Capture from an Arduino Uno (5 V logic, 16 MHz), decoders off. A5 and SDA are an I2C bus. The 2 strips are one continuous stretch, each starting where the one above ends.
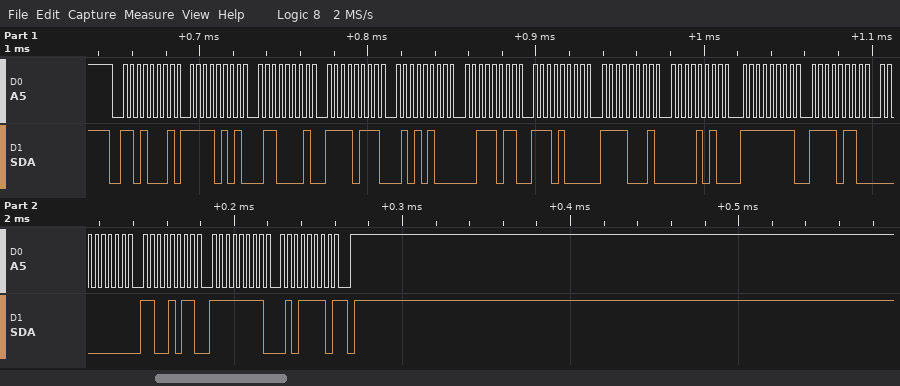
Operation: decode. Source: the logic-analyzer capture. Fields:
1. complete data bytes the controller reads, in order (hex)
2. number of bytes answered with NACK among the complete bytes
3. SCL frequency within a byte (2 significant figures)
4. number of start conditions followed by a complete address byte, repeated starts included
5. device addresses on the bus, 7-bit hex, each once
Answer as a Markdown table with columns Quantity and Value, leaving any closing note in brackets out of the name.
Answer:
| Quantity | Value |
|---|---|
| complete data bytes the controller reads, in order | F5 61 F7 54 3B E8 F1 0A FF F6 00 CB FF 5E |
| number of bytes answered with NACK among the complete bytes | 1 |
| SCL frequency within a byte | 250 kHz |
| number of start conditions followed by a complete address byte, repeated starts included | 1 |
| device addresses on the bus, 7-bit hex, each once | 0x68 |
